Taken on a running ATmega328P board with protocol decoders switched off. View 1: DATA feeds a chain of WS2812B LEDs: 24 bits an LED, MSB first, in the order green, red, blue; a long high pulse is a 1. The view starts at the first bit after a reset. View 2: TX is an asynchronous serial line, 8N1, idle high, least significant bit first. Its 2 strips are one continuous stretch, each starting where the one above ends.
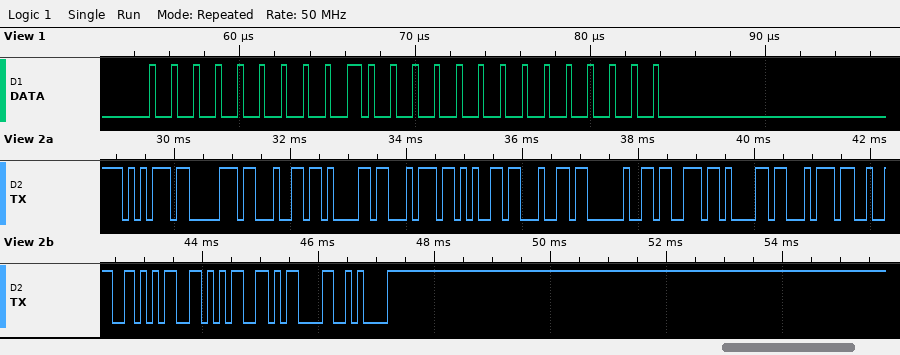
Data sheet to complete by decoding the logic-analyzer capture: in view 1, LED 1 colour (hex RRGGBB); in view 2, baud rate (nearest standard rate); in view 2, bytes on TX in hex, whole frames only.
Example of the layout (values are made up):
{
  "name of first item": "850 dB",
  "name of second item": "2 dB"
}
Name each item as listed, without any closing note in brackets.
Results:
{
  "in view 1, LED 1 colour": "#400000",
  "in view 2, baud rate": "9600 baud",
  "in view 2, bytes on TX in hex, whole frames only": "75 70 64 61 74 65 64 20 73 61 74 32 35 35 0D 0A"
}
